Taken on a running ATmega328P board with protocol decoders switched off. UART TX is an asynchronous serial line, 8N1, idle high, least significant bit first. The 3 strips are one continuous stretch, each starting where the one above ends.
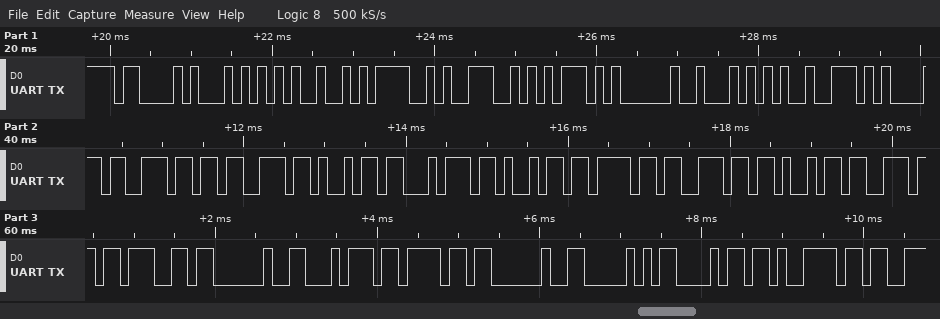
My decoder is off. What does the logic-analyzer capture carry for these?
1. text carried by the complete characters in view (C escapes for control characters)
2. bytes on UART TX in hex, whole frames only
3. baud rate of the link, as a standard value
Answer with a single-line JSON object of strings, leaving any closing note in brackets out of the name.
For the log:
{"text carried by the complete characters in view": "\"CTION] Transitioning to Phy\"", "bytes on UART TX in hex, whole frames only": "0x43 0x54 0x49 0x4F 0x4E 0x5D 0x20 0x54 0x72 0x61 0x6E 0x73 0x69 0x74 0x69 0x6F 0x6E 0x69 0x6E 0x67 0x20 0x74 0x6F 0x20 0x50 0x68 0x79", "baud rate of the link, as a standard value": "9600 baud"}
